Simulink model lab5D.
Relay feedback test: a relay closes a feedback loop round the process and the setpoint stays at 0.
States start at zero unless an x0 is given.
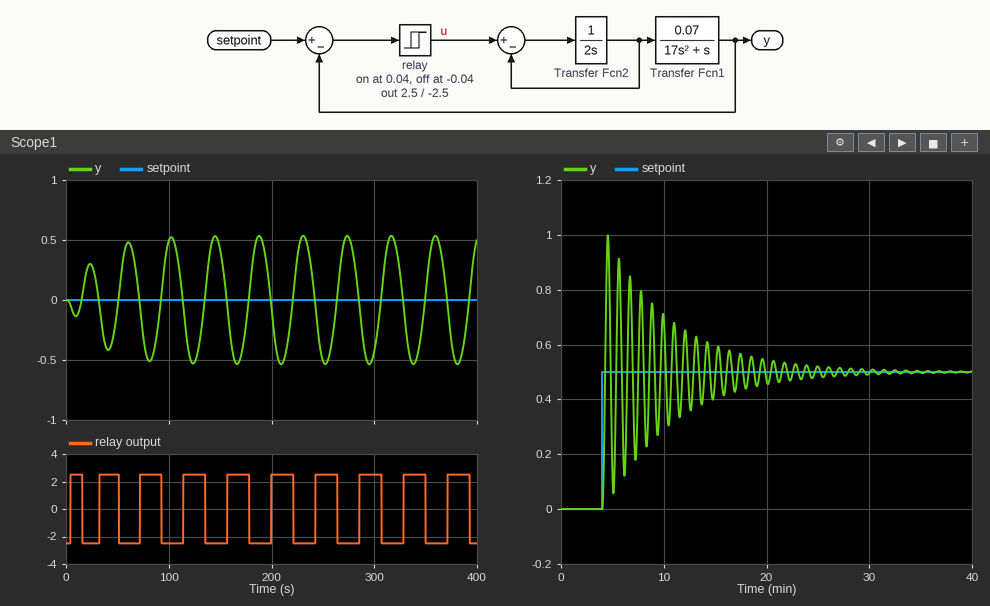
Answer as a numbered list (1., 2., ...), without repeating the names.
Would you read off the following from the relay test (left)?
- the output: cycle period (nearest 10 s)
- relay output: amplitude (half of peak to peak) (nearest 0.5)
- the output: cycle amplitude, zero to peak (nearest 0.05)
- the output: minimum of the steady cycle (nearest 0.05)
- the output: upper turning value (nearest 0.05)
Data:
1. 40 s
2. 2.5
3. 0.55
4. -0.55
5. 0.55
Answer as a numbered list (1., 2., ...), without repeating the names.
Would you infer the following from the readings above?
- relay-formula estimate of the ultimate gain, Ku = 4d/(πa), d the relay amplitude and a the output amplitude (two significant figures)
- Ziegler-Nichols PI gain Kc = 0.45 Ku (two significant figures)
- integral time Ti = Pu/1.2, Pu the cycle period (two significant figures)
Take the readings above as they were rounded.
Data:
1. 5.8
2. 2.6
3. 33 s
